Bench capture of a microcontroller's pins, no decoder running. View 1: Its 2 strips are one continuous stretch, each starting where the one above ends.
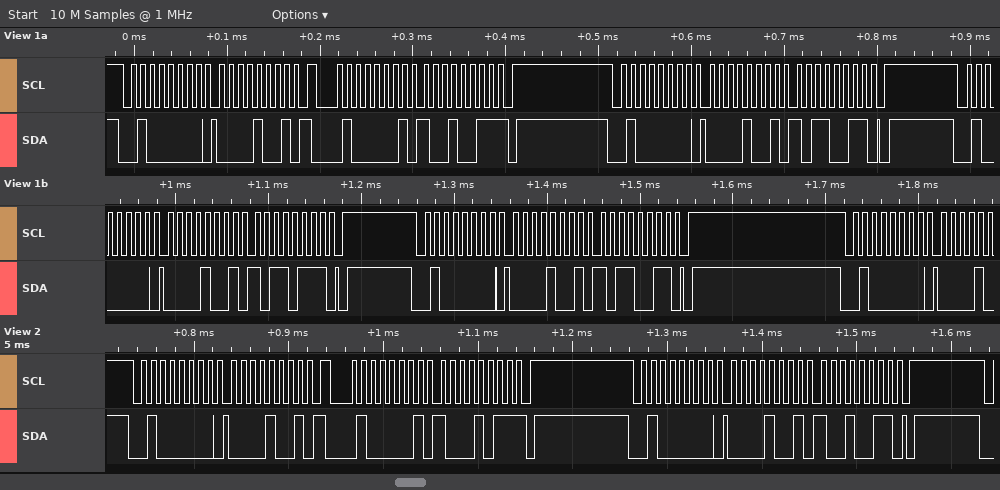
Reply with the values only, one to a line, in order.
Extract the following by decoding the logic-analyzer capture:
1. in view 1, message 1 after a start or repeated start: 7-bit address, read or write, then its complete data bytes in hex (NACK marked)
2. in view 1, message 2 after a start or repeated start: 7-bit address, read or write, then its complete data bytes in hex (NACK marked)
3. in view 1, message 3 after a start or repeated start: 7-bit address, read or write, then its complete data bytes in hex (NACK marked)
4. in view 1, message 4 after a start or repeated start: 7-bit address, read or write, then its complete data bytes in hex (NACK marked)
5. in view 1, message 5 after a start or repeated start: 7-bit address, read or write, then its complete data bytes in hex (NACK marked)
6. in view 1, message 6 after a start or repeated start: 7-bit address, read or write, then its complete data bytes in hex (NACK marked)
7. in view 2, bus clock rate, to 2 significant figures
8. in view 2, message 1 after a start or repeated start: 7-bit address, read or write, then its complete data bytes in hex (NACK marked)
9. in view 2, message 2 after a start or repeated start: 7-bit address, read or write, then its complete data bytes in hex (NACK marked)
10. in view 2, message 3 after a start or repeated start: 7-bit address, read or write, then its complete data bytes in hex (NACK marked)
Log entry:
0x20 write: 09
0x20 read: 93 NACK
0x20 write: 09 B3
0x20 write: 09 B7
0x20 write: 09 B3
0x20 write
100 kHz
0x20 write: 09
0x20 read: 8B NACK
0x20 write: 09 93
